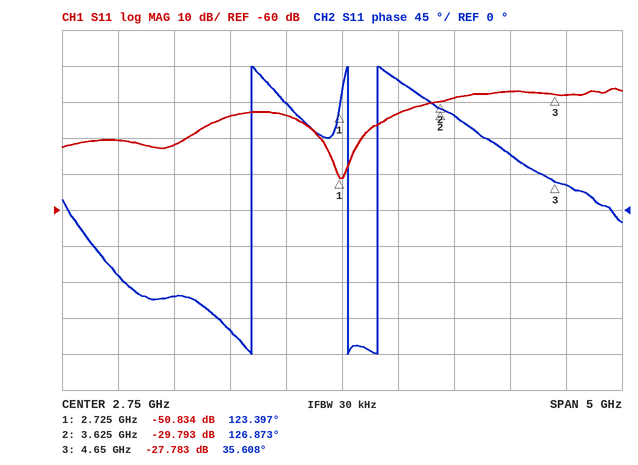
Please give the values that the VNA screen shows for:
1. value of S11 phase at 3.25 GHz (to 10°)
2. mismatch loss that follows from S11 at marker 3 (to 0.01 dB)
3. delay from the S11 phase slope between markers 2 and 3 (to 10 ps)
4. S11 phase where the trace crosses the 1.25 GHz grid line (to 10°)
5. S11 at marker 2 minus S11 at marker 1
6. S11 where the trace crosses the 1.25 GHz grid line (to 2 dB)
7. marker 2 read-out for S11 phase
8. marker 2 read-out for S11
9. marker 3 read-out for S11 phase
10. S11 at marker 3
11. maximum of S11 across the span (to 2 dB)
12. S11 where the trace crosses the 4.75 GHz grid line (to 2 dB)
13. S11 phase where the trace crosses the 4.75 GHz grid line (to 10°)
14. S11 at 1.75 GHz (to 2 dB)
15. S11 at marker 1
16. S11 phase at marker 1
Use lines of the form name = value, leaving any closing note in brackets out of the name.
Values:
value of S11 phase at 3.25 GHz = 160°
mismatch loss that follows from S11 at marker 3 = 0.01 dB
delay from the S11 phase slope between markers 2 and 3 = 250 ps
S11 phase where the trace crosses the 1.25 GHz grid line = -110°
S11 at marker 2 minus S11 at marker 1 = 21.041 dB
S11 where the trace crosses the 1.25 GHz grid line = -42 dB
marker 2 read-out for S11 phase = 126.873°
marker 2 read-out for S11 = -29.793 dB
marker 3 read-out for S11 phase = 35.608°
S11 at marker 3 = -27.783 dB
maximum of S11 across the span = -26 dB
S11 where the trace crosses the 4.75 GHz grid line = -28 dB
S11 phase where the trace crosses the 4.75 GHz grid line = 30°
S11 at 1.75 GHz = -34 dB
S11 at marker 1 = -50.834 dB
S11 phase at marker 1 = 123.397°
